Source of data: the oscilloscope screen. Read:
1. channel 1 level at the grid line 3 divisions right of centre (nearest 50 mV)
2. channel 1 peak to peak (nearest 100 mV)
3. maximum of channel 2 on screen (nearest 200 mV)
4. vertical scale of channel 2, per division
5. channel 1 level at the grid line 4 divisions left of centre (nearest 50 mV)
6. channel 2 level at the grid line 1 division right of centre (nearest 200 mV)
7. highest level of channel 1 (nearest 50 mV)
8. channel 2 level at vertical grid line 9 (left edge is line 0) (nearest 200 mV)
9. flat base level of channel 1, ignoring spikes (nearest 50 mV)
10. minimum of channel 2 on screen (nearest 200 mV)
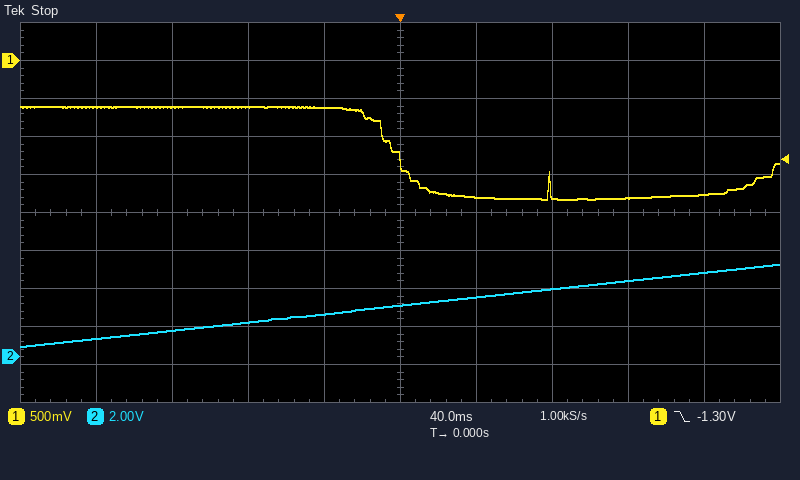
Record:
-1.80 V
1.20 V
4.8 V
2 V
-600 mV
3.2 V
-600 mV
4.4 V
-1.80 V
600 mV
